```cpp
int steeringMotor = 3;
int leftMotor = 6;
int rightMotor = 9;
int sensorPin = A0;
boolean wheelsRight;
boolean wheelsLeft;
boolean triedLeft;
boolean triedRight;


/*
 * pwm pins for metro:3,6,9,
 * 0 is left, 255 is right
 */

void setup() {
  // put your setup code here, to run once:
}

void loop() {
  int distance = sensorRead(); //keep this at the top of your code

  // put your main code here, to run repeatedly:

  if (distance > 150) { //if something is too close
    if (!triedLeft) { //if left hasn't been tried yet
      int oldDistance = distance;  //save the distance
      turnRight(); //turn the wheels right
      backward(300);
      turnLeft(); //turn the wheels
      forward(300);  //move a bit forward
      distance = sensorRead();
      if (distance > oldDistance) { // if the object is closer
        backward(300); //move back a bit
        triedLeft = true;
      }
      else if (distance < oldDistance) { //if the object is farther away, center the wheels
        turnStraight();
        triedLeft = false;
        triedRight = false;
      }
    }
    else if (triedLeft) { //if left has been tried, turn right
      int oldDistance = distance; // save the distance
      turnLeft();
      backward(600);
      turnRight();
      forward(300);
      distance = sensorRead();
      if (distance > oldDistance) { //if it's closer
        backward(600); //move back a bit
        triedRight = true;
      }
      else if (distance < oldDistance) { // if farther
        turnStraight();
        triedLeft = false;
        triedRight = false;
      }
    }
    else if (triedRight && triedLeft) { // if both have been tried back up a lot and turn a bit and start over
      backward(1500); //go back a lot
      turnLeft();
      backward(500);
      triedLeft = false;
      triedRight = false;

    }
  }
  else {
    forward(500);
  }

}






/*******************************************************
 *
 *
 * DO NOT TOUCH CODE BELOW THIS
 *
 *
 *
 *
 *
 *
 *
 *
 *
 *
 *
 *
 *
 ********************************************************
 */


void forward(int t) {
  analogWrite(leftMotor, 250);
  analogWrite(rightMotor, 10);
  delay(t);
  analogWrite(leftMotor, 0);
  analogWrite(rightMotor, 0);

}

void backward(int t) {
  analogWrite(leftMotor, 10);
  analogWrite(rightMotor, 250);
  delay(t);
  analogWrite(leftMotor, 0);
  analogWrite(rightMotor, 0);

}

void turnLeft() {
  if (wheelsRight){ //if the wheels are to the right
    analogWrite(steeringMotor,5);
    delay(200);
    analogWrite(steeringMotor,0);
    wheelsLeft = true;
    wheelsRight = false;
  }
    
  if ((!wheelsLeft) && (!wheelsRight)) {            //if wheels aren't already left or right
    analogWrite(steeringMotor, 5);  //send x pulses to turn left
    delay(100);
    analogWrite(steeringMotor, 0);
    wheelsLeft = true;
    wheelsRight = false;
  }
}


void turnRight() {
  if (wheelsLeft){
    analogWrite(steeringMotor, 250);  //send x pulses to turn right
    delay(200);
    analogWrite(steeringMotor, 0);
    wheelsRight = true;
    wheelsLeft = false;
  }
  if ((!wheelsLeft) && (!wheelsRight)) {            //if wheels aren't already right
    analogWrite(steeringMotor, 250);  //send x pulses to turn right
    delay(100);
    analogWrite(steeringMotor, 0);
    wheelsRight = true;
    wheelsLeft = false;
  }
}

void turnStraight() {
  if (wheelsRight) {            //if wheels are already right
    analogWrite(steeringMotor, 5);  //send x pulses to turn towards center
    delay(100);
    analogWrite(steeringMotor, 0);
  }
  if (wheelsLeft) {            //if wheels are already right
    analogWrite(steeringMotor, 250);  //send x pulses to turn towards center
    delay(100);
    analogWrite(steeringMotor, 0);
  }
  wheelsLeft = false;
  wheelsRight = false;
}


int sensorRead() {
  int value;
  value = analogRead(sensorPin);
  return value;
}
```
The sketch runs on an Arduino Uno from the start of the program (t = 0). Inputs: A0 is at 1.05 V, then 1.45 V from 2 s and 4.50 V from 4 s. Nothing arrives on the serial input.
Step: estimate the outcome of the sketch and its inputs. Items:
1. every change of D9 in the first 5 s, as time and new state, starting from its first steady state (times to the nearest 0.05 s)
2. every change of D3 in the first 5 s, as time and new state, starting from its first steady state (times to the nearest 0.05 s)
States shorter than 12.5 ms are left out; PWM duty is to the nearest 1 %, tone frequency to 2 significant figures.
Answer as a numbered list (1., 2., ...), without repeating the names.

1. 0.1 s PWM 98 %; 0.4 s low; 0.6 s PWM 4 %; 0.9 s low; 1.1 s PWM 98 %; 1.4 s low; 1.6 s PWM 4 %; 1.9 s low; 2.1 s PWM 98 %; 2.4 s low; 2.6 s PWM 4 %; 2.9 s PWM 98 %; 3.8 s low; 4 s PWM 4 %; 4.3 s PWM 98 %; 4.9 s low
2. 0 s PWM 98 %; 0.1 s low; 0.4 s PWM 2 %; 0.6 s low; 0.9 s PWM 98 %; 1.1 s low; 1.4 s PWM 2 %; 1.6 s low; 1.9 s PWM 98 %; 2.1 s low; 2.4 s PWM 2 %; 2.6 s low; 3.8 s PWM 98 %; 4 s low; 4.9 s PWM 2 %
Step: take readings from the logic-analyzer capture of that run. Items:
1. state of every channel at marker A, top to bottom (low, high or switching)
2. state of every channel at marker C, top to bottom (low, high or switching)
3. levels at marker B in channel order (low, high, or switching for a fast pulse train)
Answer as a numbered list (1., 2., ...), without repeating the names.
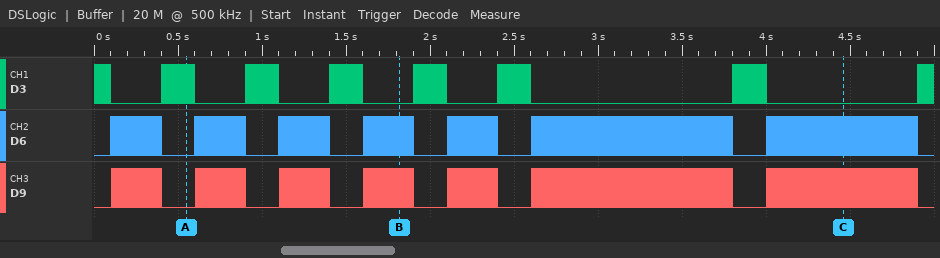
1. D3 switching, D6 low, D9 low
2. D3 low, D6 switching, D9 switching
3. D3 low, D6 switching, D9 switching
